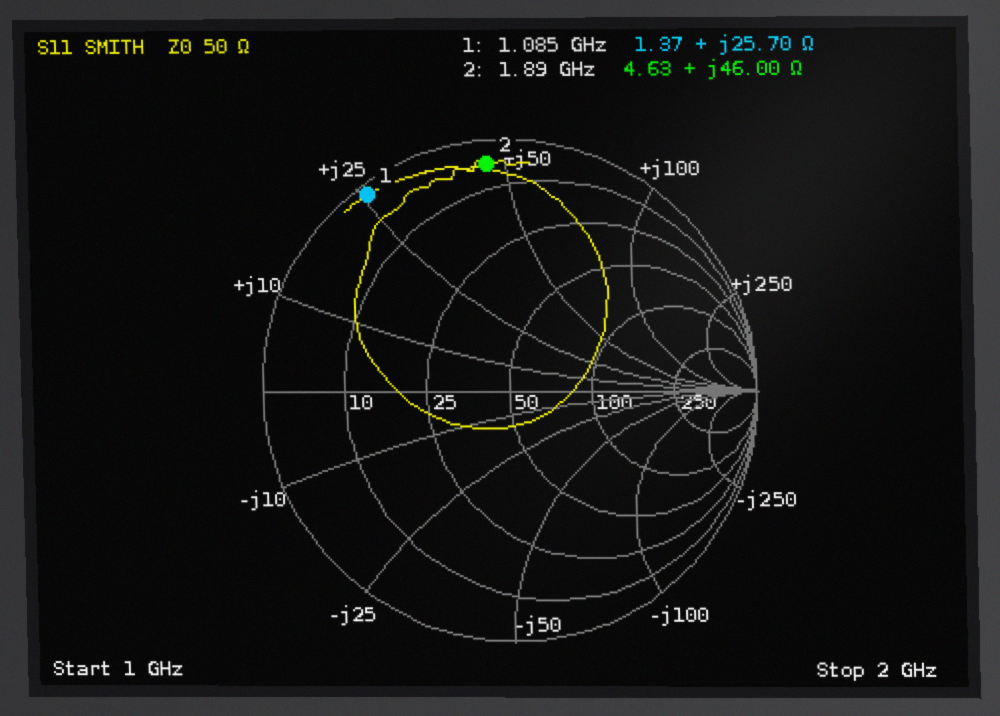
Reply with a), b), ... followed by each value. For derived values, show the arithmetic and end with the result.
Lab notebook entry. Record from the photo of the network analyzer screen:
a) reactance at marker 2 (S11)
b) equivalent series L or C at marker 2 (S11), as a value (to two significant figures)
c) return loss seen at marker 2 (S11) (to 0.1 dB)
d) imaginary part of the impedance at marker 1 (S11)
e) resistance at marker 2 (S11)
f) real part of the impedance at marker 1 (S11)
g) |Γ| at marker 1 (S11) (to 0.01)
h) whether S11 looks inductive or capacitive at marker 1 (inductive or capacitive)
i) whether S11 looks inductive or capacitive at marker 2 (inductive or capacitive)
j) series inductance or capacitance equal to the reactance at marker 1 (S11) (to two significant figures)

a) +46.00 Ω
b) L = 46 Ω/(2π × 1.89 GHz) ≈ 3.9 nH
c) 0.9 dB
d) +25.70 Ω
e) 4.63 Ω
f) 1.37 Ω
g) 0.96
h) inductive
i) inductive
j) L = 25.7 Ω/(2π × 1.085 GHz) ≈ 3.8 nH
